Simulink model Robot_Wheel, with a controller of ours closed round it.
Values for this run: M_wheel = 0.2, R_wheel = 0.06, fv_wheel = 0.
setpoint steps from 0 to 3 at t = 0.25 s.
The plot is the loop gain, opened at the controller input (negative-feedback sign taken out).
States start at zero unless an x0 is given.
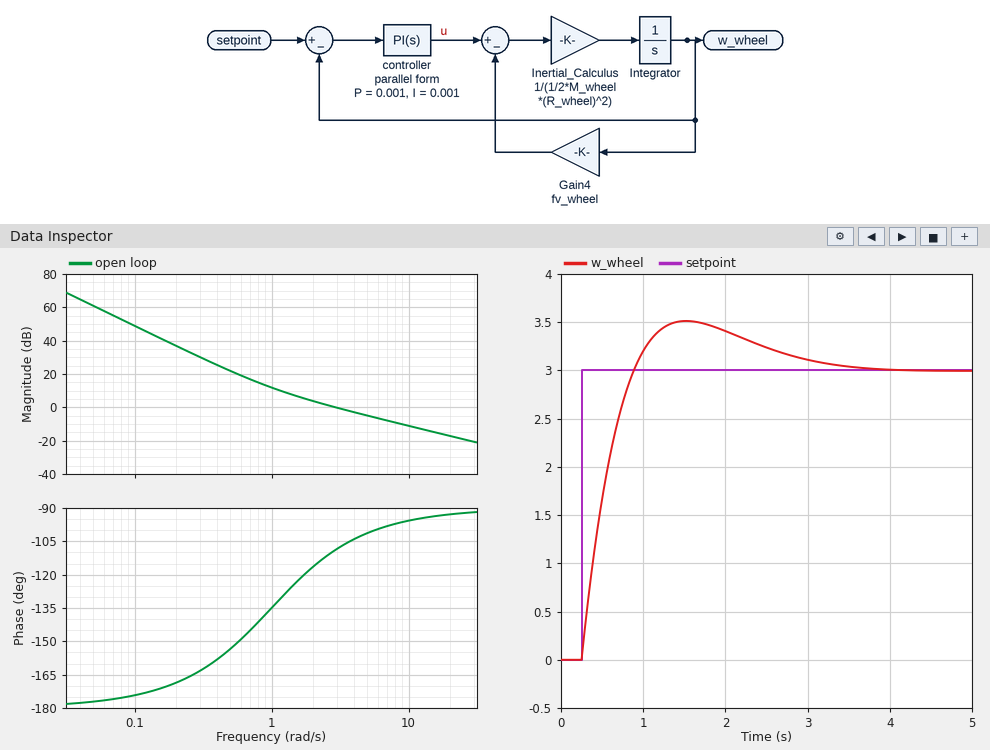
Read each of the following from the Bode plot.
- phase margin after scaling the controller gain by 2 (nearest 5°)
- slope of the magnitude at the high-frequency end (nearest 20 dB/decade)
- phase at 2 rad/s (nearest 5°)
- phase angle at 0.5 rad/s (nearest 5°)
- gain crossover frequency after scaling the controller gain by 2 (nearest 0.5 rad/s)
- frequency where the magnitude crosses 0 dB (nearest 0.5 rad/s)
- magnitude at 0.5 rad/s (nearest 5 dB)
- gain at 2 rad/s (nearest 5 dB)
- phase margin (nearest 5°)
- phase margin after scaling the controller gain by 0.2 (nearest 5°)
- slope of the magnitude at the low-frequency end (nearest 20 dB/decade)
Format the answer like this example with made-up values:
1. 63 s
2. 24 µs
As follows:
1. 80°
2. -20 dB/decade
3. -115°
4. -155°
5. 5.5 rad/s
6. 3.0 rad/s
7. 20 dB
8. 5 dB
9. 70°
10. 40°
11. -40 dB/decade
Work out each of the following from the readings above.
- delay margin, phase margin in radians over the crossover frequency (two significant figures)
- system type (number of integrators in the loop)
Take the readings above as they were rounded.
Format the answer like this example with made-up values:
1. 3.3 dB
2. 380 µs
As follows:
1. 0.41 s
2. 2
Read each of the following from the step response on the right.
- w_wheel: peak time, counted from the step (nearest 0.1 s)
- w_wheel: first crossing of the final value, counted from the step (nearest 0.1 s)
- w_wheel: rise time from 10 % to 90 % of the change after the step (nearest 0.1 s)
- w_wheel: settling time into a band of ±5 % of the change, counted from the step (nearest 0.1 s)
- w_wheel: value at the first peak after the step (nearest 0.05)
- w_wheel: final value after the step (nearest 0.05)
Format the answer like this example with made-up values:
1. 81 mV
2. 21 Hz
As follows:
1. 1.3 s
2. 0.6 s
3. 0.5 s
4. 2.6 s
5. 3.50
6. 3.00
